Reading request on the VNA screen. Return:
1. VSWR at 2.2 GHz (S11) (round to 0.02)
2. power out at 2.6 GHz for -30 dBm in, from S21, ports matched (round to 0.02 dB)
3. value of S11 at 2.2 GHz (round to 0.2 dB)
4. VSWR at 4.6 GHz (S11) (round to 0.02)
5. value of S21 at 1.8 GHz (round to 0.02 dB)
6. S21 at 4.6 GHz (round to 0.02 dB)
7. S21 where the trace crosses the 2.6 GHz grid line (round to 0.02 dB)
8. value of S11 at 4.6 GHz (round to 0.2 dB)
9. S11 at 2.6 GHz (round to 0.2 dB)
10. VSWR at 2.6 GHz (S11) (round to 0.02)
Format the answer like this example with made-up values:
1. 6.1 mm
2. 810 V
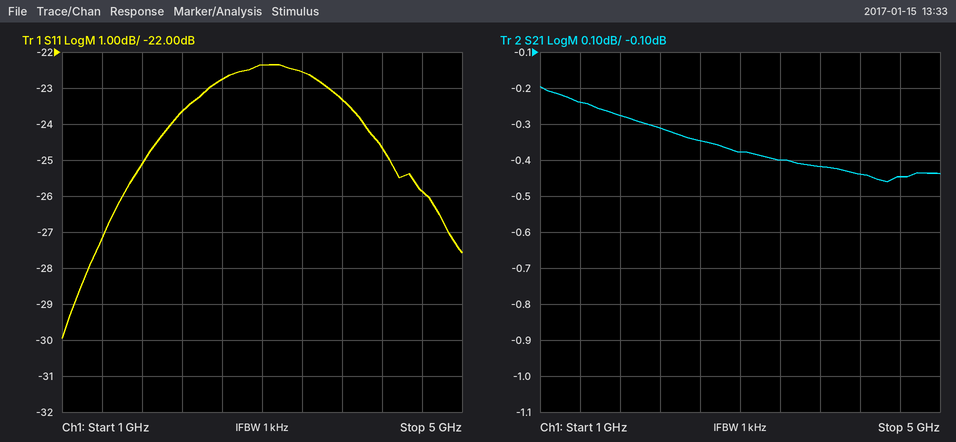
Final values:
1. 1.14
2. -30.34 dBm
3. -23.6 dB
4. 1.10
5. -0.28 dB
6. -0.44 dB
7. -0.34 dB
8. -25.8 dB
9. -22.8 dB
10. 1.16
